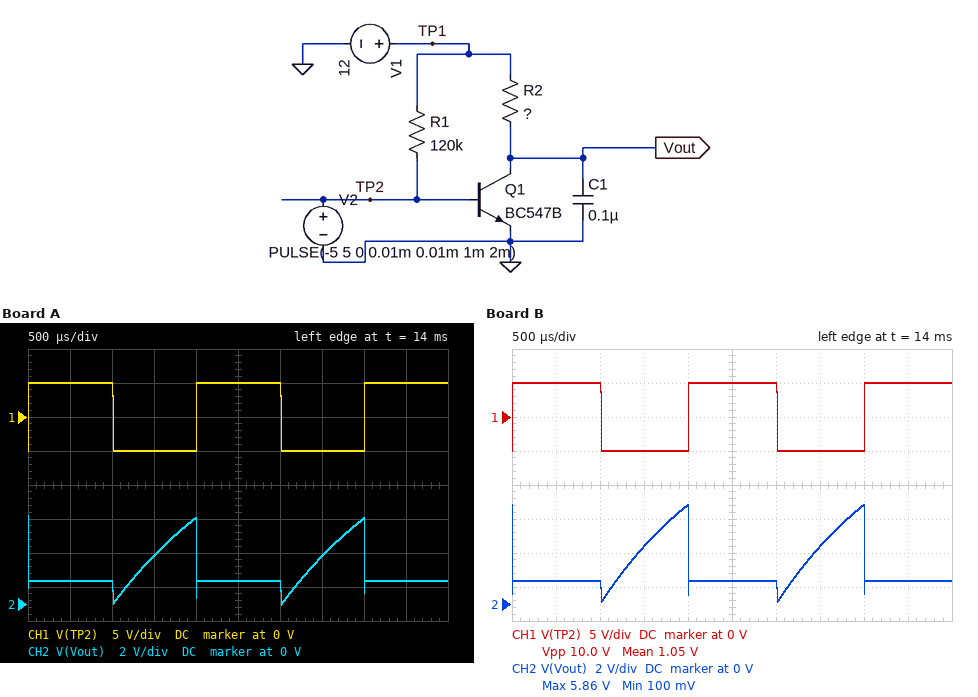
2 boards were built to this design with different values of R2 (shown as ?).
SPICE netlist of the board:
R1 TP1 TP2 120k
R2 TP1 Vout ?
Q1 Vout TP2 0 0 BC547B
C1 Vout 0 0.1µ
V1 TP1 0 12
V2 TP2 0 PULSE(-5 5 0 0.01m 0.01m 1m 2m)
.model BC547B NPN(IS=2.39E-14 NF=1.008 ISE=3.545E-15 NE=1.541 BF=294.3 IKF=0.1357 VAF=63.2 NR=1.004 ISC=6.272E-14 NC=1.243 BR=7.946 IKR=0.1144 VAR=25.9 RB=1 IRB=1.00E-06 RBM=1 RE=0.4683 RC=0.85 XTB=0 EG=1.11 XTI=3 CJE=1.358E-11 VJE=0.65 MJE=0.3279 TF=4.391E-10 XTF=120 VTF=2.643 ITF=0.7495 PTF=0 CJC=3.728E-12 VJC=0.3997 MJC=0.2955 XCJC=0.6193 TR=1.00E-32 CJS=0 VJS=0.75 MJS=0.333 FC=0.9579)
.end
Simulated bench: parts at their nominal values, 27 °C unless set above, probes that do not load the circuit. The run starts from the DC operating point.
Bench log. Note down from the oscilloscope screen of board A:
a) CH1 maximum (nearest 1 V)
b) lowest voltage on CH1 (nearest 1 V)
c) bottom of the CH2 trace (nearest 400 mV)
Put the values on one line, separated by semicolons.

5 V; -5 V; 0 V
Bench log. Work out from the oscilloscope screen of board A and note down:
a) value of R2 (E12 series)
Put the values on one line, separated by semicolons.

18 kΩ
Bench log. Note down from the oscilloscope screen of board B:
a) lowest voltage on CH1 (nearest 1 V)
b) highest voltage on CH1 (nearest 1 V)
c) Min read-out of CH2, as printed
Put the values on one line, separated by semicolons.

-5 V; 5 V; 100 mV
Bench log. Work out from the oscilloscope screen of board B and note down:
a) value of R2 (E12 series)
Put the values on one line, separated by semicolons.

15 kΩ
